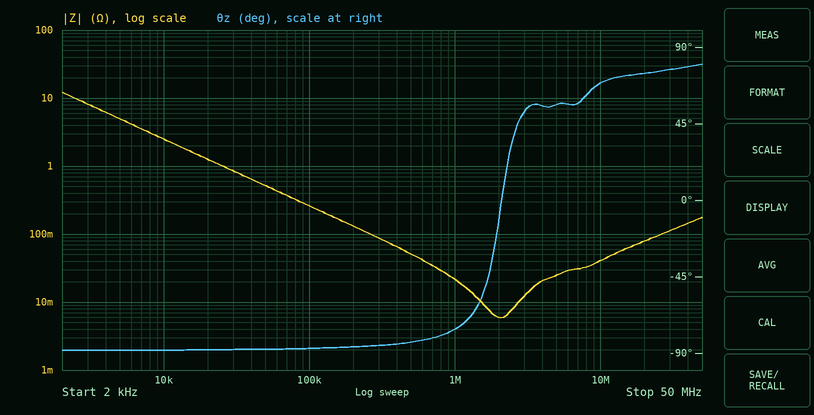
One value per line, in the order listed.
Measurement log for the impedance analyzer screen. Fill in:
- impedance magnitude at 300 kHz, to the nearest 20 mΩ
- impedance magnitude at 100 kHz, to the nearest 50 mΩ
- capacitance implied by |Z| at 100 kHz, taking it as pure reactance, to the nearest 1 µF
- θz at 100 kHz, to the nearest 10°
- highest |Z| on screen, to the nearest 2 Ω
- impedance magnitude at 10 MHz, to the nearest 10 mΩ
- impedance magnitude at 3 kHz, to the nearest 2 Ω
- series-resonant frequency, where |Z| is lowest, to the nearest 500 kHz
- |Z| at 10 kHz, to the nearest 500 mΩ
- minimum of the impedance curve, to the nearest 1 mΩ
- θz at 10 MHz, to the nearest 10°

80 mΩ
250 mΩ
6 µF
-90°
12 Ω
40 mΩ
8 Ω
2.0 MHz
2.5 Ω
6 mΩ
70°
